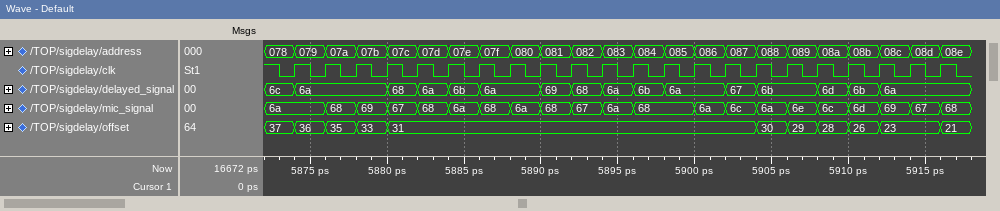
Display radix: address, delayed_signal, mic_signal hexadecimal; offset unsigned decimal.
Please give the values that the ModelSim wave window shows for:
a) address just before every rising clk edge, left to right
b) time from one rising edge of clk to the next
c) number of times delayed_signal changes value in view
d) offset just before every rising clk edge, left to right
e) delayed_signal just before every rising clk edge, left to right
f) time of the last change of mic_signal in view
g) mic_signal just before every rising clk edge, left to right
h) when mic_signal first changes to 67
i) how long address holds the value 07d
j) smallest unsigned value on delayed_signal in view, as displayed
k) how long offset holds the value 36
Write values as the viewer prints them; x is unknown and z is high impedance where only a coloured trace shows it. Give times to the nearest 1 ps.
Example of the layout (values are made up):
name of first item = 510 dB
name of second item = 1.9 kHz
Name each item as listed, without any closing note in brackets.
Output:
address just before every rising clk edge, left to right = 078, 079, 07a, 07b, 07c, 07d, 07e, 07f, 080, 081, 082, 083, 084, 085, 086, 087, 088, 089, 08a, 08b, 08c, 08d
time from one rising edge of clk to the next = 2 ps
number of times delayed_signal changes value in view = 15
offset just before every rising clk edge, left to right = 37, 36, 35, 33, 31, 31, 31, 31, 31, 31, 31, 31, 31, 31, 31, 31, 30, 29, 28, 26, 23, 23
delayed_signal just before every rising clk edge, left to right = 6c, 6a, 6a, 6a, 68, 6a, 6b, 6a, 6a, 69, 68, 6a, 6b, 6a, 6a, 67, 6b, 6b, 6d, 6b, 6a, 6a
time of the last change of mic_signal in view = 5916 ps
mic_signal just before every rising clk edge, left to right = 6a, 6a, 68, 69, 67, 68, 6a, 68, 6a, 68, 67, 6a, 68, 68, 6a, 6c, 6a, 6e, 6c, 6d, 69, 67
when mic_signal first changes to 67 = 5880 ps
how long address holds the value 07d = 2 ps
smallest unsigned value on delayed_signal in view, as displayed = 67
how long offset holds the value 36 = 2 ps
